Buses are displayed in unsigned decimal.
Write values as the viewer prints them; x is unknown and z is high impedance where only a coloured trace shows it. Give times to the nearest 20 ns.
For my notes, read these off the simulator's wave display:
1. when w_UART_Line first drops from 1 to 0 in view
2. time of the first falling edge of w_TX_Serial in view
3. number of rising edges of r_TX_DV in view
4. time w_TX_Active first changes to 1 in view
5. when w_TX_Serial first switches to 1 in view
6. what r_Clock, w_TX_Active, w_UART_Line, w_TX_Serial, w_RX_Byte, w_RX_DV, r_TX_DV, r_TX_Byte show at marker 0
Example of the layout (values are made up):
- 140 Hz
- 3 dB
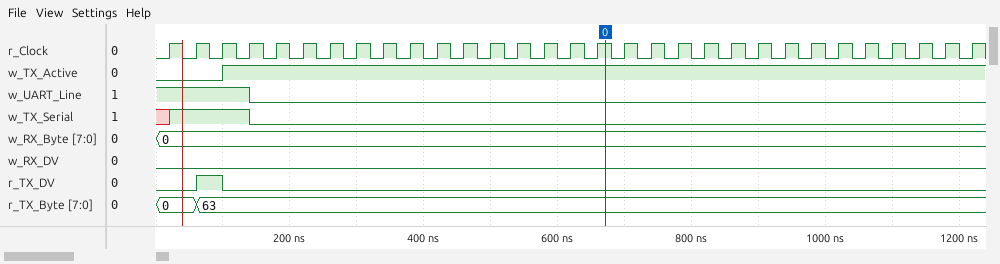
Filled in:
- 140 ns
- 140 ns
- 1
- 100 ns
- 20 ns
- r_Clock=1, w_TX_Active=1, w_UART_Line=0, w_TX_Serial=0, w_RX_Byte=0, w_RX_DV=0, r_TX_DV=0, r_TX_Byte=63
